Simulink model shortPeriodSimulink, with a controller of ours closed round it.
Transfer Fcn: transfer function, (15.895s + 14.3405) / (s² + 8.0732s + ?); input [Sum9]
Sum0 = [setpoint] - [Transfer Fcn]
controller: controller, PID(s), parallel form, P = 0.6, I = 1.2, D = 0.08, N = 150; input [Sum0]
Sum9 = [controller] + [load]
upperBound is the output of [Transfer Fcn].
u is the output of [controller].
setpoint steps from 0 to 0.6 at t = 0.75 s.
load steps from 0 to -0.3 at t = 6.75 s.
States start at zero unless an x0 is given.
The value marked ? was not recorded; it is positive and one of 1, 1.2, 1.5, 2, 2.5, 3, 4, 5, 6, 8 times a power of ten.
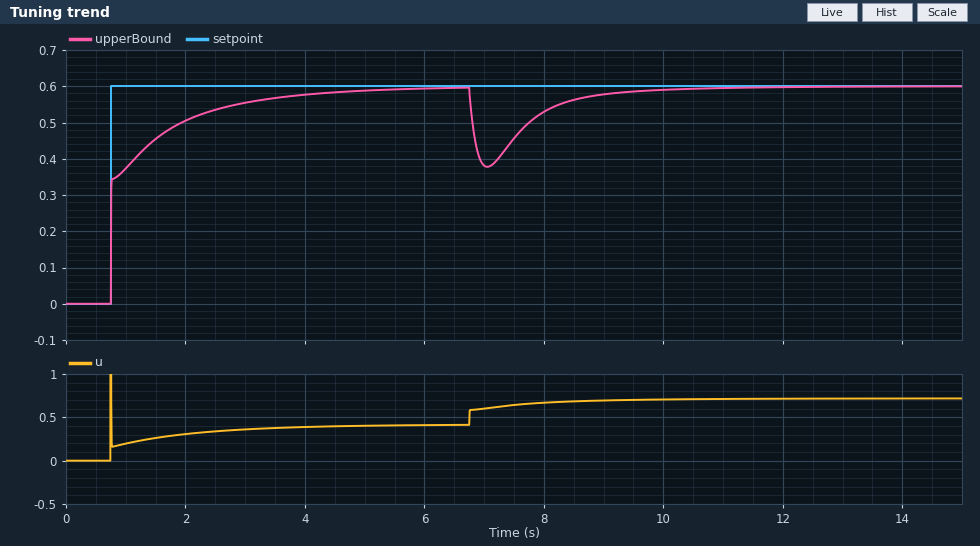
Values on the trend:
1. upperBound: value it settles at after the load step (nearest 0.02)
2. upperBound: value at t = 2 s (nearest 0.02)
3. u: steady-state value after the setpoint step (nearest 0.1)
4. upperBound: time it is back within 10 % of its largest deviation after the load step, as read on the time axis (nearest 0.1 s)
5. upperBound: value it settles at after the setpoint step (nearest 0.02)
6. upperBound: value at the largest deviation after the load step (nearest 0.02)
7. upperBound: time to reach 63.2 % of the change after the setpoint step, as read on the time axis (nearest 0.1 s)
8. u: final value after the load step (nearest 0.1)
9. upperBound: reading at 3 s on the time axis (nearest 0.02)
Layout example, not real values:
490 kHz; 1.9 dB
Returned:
0.60; 0.50; 0.4; 9.0 s; 0.60; 0.38; 1.0 s; 0.7; 0.56
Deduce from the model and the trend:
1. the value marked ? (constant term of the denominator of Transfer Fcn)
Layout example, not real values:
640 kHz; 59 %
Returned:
10
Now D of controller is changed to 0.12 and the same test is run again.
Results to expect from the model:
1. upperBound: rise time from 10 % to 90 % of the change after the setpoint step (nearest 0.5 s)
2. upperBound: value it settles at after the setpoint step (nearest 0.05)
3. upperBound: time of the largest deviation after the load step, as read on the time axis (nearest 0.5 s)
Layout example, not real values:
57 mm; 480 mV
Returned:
2.0 s; 0.60; 7.0 s
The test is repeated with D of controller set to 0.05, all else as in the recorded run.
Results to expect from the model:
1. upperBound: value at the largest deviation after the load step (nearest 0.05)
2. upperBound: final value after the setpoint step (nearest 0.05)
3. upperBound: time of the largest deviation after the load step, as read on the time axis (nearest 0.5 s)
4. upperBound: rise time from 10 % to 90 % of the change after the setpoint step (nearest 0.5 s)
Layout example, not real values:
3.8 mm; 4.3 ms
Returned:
0.35; 0.60; 7.0 s; 2.0 s
